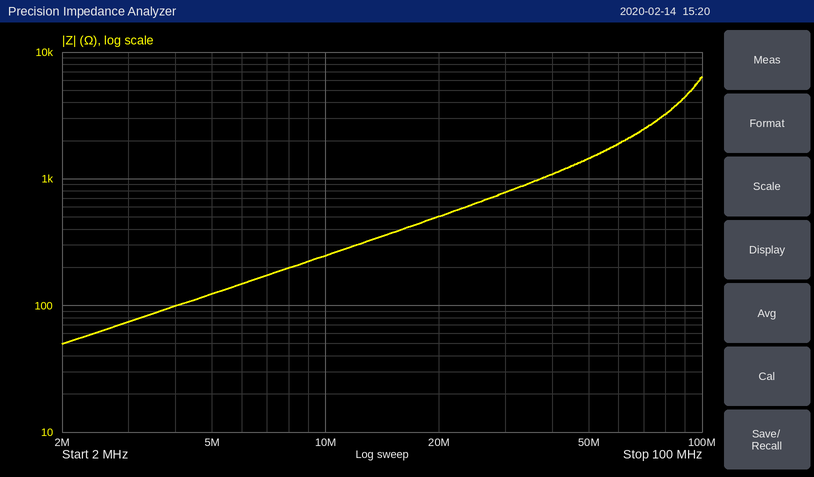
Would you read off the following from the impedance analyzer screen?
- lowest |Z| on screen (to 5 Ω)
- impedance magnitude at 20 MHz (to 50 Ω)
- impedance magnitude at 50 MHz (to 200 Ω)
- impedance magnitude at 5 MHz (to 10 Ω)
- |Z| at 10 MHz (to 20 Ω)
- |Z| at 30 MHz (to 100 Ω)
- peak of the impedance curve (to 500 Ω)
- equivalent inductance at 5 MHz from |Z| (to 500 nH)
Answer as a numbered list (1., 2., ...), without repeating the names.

1. 50 Ω
2. 500 Ω
3. 1.4 kΩ
4. 120 Ω
5. 240 Ω
6. 800 Ω
7. 6.5 kΩ
8. 4.0 µH
